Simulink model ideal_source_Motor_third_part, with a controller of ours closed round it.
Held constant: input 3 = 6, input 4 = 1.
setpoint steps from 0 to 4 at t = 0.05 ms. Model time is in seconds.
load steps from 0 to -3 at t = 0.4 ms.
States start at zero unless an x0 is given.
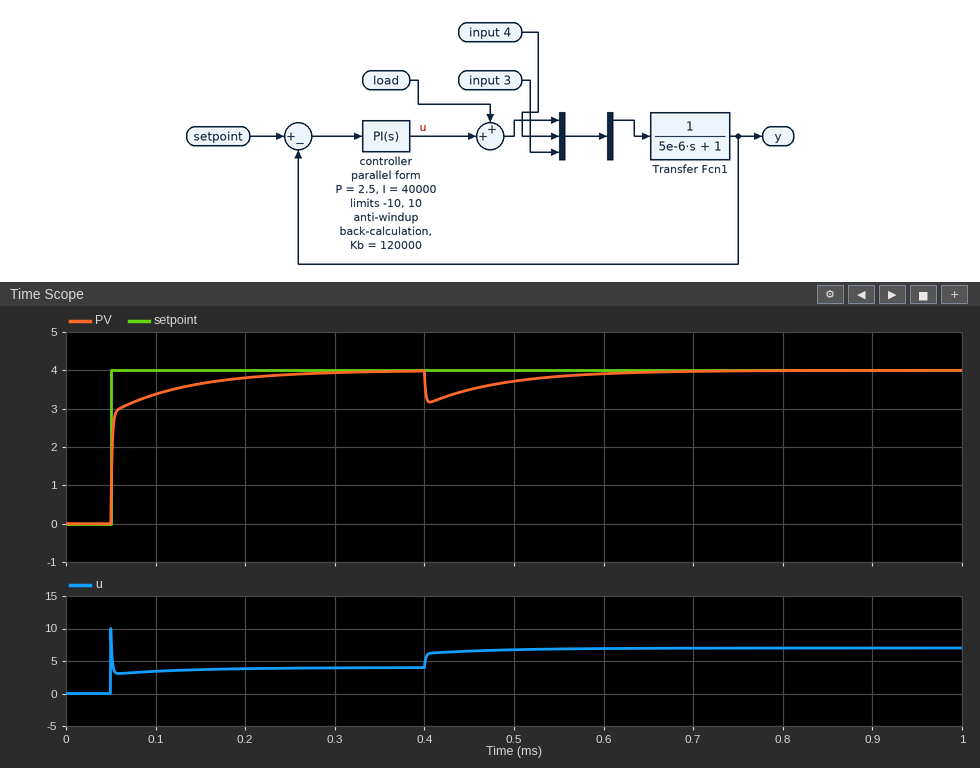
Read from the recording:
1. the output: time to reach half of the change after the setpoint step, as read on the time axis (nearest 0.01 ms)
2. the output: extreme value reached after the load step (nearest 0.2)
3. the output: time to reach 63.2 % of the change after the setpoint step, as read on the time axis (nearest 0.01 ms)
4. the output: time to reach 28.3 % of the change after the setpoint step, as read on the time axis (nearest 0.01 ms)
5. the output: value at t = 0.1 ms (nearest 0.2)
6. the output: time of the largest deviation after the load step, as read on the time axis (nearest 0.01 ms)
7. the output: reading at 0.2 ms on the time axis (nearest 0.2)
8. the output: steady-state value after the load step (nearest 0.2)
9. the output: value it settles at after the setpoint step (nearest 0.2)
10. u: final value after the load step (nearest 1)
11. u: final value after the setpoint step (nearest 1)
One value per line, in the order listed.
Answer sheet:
0.05 ms
3.2
0.05 ms
0.05 ms
3.4
0.41 ms
3.8
4.0
4.0
7
4
